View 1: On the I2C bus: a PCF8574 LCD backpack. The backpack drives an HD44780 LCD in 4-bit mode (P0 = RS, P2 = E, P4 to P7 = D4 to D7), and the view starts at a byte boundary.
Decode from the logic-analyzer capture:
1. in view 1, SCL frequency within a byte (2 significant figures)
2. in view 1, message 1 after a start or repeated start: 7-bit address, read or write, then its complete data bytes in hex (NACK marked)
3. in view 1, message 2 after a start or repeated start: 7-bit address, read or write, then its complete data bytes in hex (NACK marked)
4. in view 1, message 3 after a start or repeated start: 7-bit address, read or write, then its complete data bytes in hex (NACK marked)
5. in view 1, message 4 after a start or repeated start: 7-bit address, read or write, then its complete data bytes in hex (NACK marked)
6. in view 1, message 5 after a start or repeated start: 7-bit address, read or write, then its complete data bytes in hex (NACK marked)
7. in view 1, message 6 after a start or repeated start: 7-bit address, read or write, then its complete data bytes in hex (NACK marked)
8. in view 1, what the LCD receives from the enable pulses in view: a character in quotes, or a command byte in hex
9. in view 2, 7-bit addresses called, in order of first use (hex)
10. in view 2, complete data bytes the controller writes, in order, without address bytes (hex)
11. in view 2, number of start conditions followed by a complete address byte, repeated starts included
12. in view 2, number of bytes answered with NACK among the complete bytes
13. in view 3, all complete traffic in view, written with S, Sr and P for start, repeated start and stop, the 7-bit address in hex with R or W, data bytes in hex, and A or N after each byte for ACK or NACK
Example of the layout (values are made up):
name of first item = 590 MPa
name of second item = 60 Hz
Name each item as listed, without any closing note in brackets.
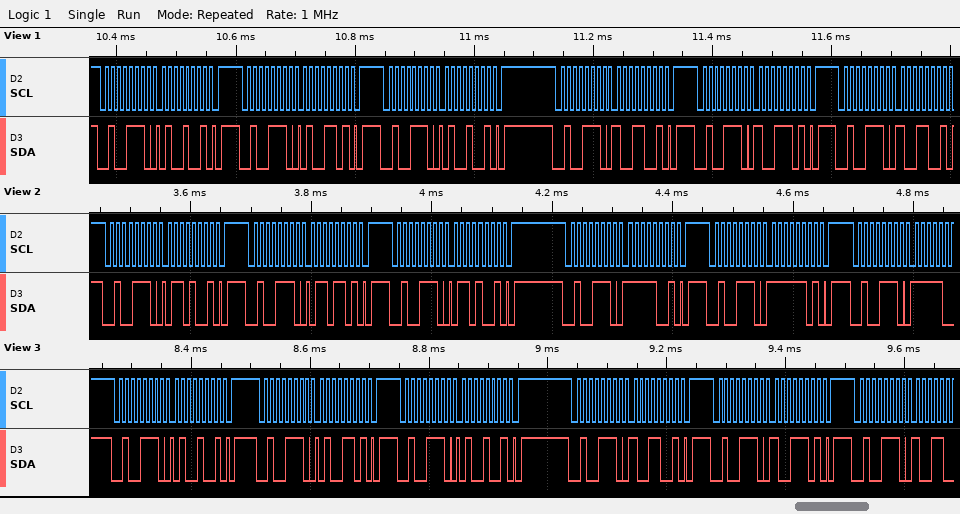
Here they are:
in view 1, SCL frequency within a byte = 100 kHz
in view 1, message 1 after a start or repeated start: 7-bit address, read or write, then its complete data bytes in hex = 0x27 write: 49
in view 1, message 2 after a start or repeated start: 7-bit address, read or write, then its complete data bytes in hex = 0x27 write: 4D
in view 1, message 3 after a start or repeated start: 7-bit address, read or write, then its complete data bytes in hex = 0x27 write: 49
in view 1, message 4 after a start or repeated start: 7-bit address, read or write, then its complete data bytes in hex = 0x27 write: 99
in view 1, message 5 after a start or repeated start: 7-bit address, read or write, then its complete data bytes in hex = 0x27 write: 9D
in view 1, message 6 after a start or repeated start: 7-bit address, read or write, then its complete data bytes in hex = 0x27 write: 99
in view 1, what the LCD receives from the enable pulses in view: a character in quotes, or a command byte in hex = 'I'
in view 2, 7-bit addresses called, in order of first use = 0x27
in view 2, complete data bytes the controller writes, in order, without address bytes = 69 6D 69 F9 FD
in view 2, number of start conditions followed by a complete address byte, repeated starts included = 6
in view 2, number of bytes answered with NACK among the complete bytes = 0
in view 3, all complete traffic in view, written with S, Sr and P for start, repeated start and stop, the 7-bit address in hex with R or W, data bytes in hex, and A or N after each byte for ACK or NACK = S 27W A 49 A P S 27W A 4D A P S 27W A 49 A P S 27W A 99 A P S 27W A 9D A P S 27W A
